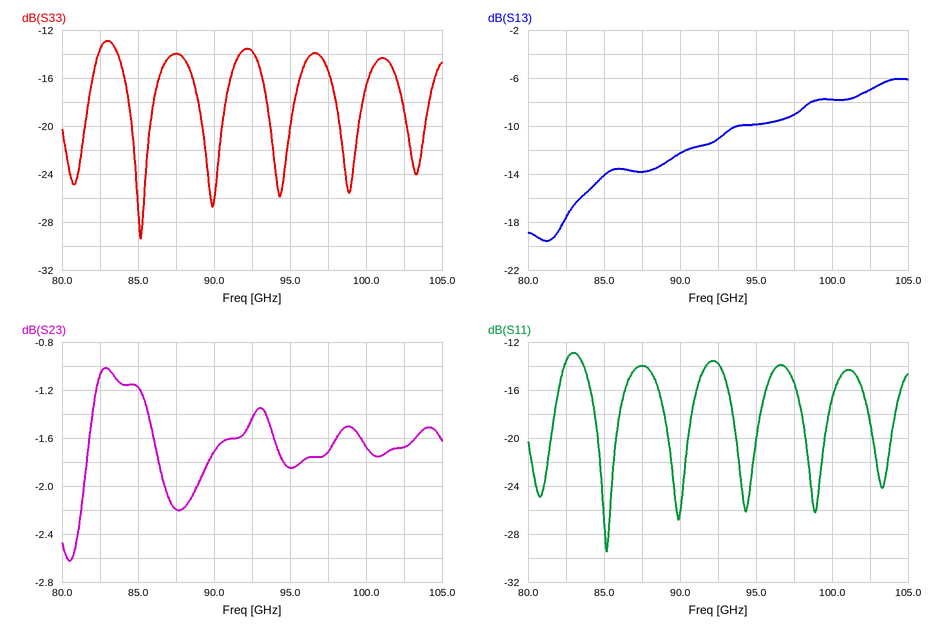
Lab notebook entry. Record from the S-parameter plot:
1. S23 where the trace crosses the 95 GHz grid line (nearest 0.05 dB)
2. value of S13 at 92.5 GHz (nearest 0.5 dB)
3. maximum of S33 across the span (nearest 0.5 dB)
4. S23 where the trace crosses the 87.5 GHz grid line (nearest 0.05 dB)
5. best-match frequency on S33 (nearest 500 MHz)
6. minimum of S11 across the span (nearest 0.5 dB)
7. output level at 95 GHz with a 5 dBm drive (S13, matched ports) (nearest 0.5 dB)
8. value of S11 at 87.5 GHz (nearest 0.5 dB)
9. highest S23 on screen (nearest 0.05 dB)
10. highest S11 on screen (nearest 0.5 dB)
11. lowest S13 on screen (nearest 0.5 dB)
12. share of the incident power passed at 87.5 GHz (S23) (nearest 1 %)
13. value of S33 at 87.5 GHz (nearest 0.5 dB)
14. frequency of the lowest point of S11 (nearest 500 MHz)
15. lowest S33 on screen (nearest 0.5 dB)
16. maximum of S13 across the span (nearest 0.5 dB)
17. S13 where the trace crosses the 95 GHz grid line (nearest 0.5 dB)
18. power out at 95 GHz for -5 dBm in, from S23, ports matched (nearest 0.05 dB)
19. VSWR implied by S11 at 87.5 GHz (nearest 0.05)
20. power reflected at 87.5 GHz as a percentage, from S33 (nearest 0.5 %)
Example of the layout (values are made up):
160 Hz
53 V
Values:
-1.85 dB
-11.0 dB
-13.0 dB
-2.20 dB
85.0 GHz
-29.5 dB
-5.0 dBm
-14.0 dB
-1.00 dB
-13.0 dB
-19.5 dB
60 %
-14.0 dB
85.0 GHz
-29.5 dB
-6.0 dB
-10.0 dB
-6.85 dBm
1.50
4.0 %
